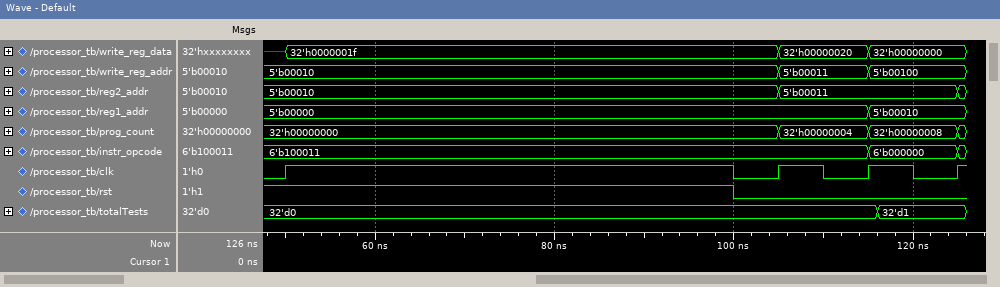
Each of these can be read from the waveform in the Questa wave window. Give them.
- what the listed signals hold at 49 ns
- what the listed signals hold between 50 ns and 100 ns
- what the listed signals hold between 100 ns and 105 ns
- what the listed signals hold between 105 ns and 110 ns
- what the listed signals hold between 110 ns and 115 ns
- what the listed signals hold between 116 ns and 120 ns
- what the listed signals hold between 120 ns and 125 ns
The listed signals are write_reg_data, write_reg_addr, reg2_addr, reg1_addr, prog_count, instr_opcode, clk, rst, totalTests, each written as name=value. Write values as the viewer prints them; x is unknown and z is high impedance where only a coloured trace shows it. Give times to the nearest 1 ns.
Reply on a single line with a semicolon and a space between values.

write_reg_data=x, write_reg_addr=5'b00010, reg2_addr=5'b00010, reg1_addr=5'b00000, prog_count=32'h00000000, instr_opcode=6'b100011, clk=0, rst=1, totalTests=32'd0; write_reg_data=32'h0000001f, write_reg_addr=5'b00010, reg2_addr=5'b00010, reg1_addr=5'b00000, prog_count=32'h00000000, instr_opcode=6'b100011, clk=1, rst=1, totalTests=32'd0; write_reg_data=32'h0000001f, write_reg_addr=5'b00010, reg2_addr=5'b00010, reg1_addr=5'b00000, prog_count=32'h00000000, instr_opcode=6'b100011, clk=0, rst=0, totalTests=32'd0; write_reg_data=32'h00000020, write_reg_addr=5'b00011, reg2_addr=5'b00011, reg1_addr=5'b00000, prog_count=32'h00000004, instr_opcode=6'b100011, clk=1, rst=0, totalTests=32'd0; write_reg_data=32'h00000020, write_reg_addr=5'b00011, reg2_addr=5'b00011, reg1_addr=5'b00000, prog_count=32'h00000004, instr_opcode=6'b100011, clk=0, rst=0, totalTests=32'd0; write_reg_data=32'h00000000, write_reg_addr=5'b00100, reg2_addr=5'b00011, reg1_addr=5'b00010, prog_count=32'h00000008, instr_opcode=6'b000000, clk=1, rst=0, totalTests=32'd1; write_reg_data=32'h00000000, write_reg_addr=5'b00100, reg2_addr=5'b00011, reg1_addr=5'b00010, prog_count=32'h00000008, instr_opcode=6'b000000, clk=0, rst=0, totalTests=32'd1
